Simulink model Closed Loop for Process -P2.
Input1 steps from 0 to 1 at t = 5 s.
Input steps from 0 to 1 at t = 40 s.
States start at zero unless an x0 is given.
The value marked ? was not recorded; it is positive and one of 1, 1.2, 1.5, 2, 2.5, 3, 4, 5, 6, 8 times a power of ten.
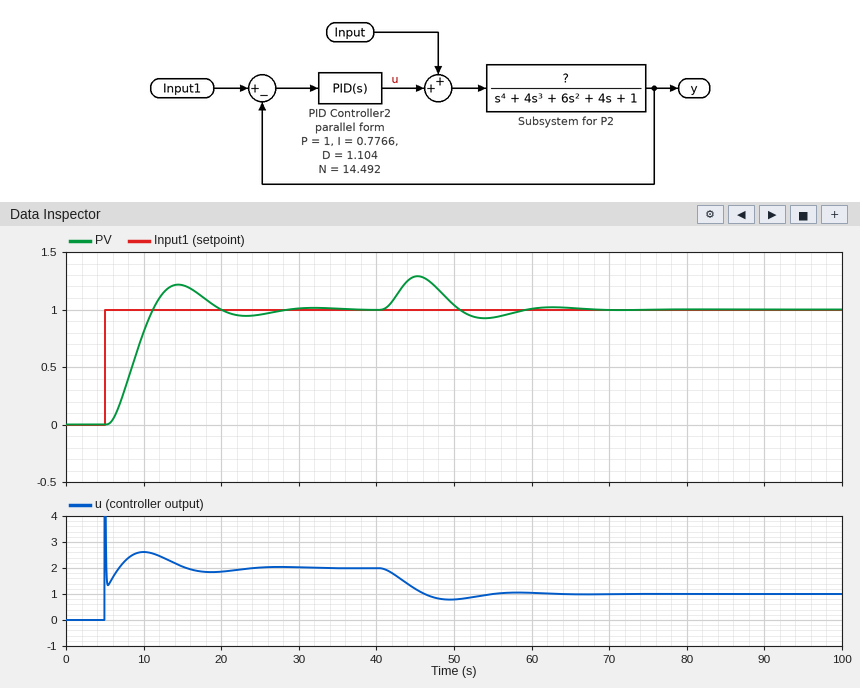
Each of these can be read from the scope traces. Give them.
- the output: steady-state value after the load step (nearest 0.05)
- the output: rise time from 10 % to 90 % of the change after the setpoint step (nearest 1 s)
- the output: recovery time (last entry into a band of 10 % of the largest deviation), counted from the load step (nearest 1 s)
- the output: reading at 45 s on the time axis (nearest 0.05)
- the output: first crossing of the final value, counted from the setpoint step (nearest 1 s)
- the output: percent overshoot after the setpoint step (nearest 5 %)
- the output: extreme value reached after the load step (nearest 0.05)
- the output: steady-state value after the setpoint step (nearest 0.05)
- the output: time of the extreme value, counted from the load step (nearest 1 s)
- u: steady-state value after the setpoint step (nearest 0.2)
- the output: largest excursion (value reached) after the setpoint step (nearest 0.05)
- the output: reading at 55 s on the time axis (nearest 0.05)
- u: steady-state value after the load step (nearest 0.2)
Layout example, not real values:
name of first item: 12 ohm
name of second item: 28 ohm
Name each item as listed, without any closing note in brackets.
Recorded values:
the output: steady-state value after the load step: 1.00
the output: rise time from 10 % to 90 % of the change after the setpoint step: 4 s
the output: recovery time (last entry into a band of 10 % of the largest deviation), counted from the load step: 18 s
the output: reading at 45 s on the time axis: 1.30
the output: first crossing of the final value, counted from the setpoint step: 6 s
the output: percent overshoot after the setpoint step: 20 %
the output: extreme value reached after the load step: 1.30
the output: steady-state value after the setpoint step: 1.00
the output: time of the extreme value, counted from the load step: 5 s
u: steady-state value after the setpoint step: 2.0
the output: largest excursion (value reached) after the setpoint step: 1.20
the output: reading at 55 s on the time axis: 0.95
u: steady-state value after the load step: 1.0
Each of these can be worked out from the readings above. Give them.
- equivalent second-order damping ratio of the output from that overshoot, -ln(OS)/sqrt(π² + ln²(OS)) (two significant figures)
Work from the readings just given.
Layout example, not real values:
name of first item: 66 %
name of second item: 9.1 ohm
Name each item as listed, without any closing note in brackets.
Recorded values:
equivalent second-order damping ratio of the output from that overshoot, -ln(OS)/sqrt(π² + ln²(OS)): 0.46
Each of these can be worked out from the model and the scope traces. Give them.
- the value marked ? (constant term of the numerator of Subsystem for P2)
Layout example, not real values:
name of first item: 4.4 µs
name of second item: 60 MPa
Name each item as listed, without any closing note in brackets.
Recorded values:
the value marked ?: 0.5
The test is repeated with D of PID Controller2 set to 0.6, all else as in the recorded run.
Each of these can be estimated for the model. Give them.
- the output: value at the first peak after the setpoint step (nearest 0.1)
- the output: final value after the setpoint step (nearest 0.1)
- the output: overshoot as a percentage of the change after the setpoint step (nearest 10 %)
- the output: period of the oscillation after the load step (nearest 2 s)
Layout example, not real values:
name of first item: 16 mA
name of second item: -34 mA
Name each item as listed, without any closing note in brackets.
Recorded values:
the output: value at the first peak after the setpoint step: 1.3
the output: final value after the setpoint step: 1.0
the output: overshoot as a percentage of the change after the setpoint step: 30 %
the output: period of the oscillation after the load step: 16 s
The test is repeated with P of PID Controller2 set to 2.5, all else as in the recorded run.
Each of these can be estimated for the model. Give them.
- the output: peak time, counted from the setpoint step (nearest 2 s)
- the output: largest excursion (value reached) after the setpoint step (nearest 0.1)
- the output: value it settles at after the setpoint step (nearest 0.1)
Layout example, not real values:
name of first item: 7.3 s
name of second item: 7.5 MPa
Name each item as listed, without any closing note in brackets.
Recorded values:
the output: peak time, counted from the setpoint step: 6 s
the output: largest excursion (value reached) after the setpoint step: 1.1
the output: value it settles at after the setpoint step: 1.0
